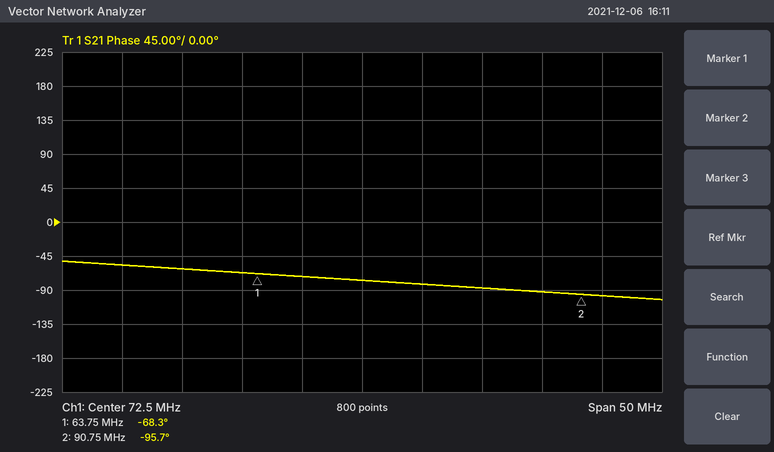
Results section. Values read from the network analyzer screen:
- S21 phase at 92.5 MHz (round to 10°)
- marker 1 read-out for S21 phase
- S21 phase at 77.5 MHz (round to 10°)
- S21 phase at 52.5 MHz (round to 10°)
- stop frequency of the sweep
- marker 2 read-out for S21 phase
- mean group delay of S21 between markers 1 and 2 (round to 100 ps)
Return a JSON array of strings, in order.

["-100°", "-68.3°", "-80°", "-60°", "97.5 MHz", "-95.7°", "2.8 ns"]
